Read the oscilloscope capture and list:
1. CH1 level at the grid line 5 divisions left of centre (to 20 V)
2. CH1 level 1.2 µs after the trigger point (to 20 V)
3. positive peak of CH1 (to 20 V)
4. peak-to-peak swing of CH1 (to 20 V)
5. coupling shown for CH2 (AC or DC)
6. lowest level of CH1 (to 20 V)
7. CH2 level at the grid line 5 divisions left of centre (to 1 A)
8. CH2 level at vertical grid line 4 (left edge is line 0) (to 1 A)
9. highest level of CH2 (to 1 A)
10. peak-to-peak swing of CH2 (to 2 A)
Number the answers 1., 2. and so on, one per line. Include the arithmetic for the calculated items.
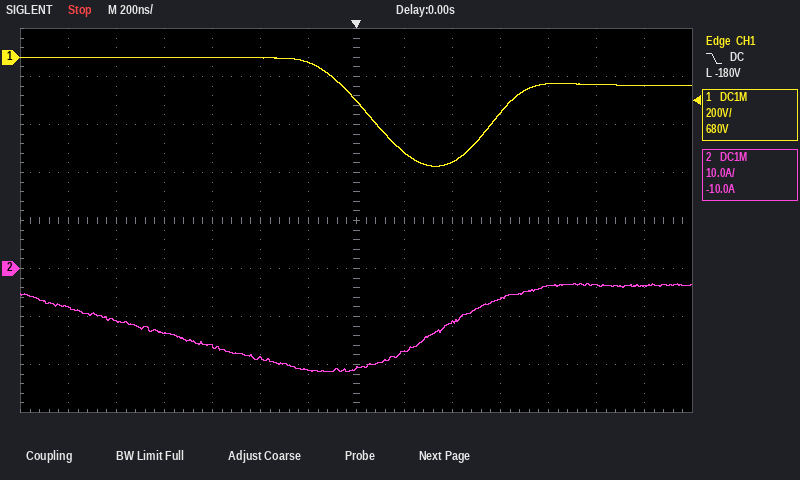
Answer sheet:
1. 0 V
2. -120 V
3. 0 V
4. 0 V − (-460 V) = 460 V
5. DC
6. -460 V
7. -11 A
8. -16 A
9. -3 A
10. 18 A
